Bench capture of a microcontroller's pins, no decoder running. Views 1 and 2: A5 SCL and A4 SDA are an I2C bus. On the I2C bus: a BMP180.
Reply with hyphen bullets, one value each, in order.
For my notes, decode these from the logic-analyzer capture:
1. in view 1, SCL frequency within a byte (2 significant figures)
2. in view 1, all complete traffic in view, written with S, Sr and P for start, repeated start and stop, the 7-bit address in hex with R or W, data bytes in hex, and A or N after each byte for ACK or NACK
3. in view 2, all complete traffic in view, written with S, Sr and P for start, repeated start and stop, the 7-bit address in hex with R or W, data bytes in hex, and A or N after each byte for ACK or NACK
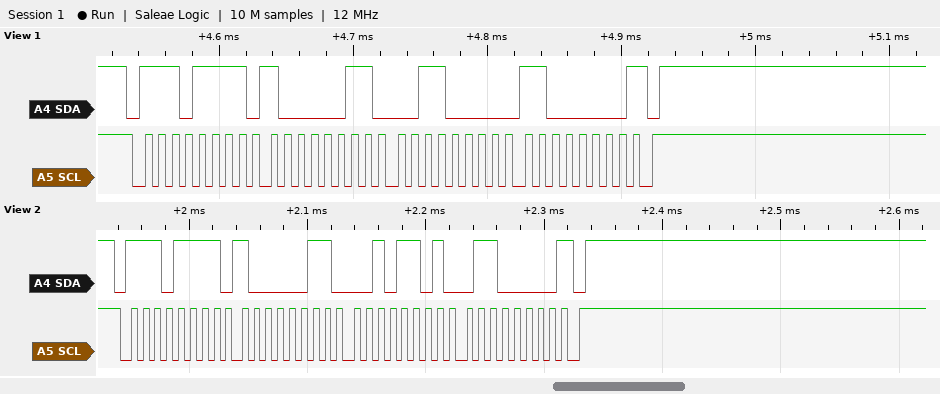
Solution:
- 100 kHz
- S 77R A 83 A 30 A C0 N P
- S 77R A 83 A 2D A 60 N P
